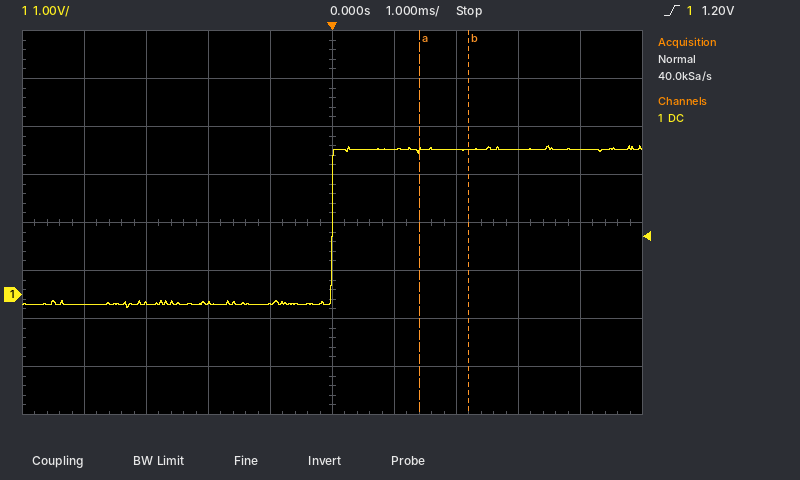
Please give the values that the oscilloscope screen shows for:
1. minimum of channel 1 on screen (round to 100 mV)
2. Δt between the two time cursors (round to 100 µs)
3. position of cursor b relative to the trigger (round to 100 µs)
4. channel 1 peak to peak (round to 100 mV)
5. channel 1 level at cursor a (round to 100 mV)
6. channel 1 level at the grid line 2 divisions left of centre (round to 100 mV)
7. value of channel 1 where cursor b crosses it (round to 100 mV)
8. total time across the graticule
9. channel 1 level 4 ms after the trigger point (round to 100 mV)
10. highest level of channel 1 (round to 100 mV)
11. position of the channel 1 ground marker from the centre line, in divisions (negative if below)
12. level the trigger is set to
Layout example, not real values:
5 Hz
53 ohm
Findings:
-300 mV
800 µs
+2.2 ms
3.4 V
3.0 V
-200 mV
3.0 V
10 ms
3.0 V
3.1 V
-1.5 div
1.20 V
